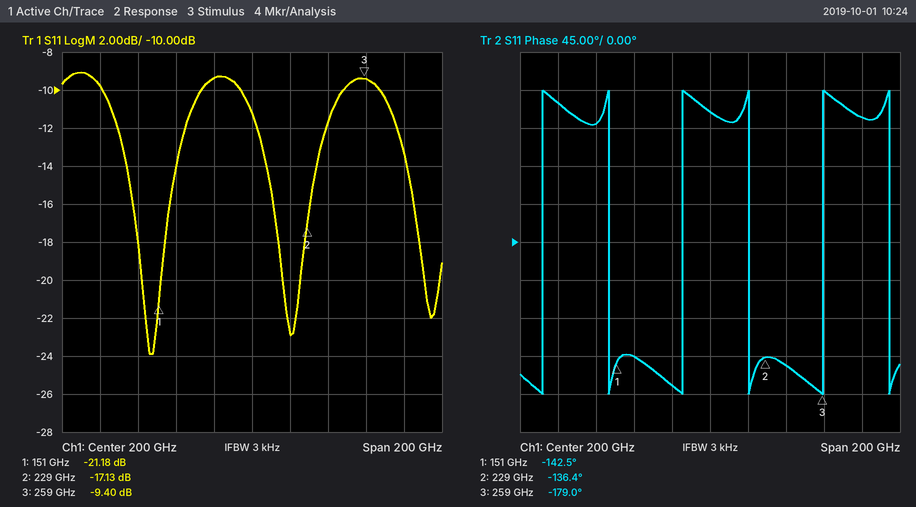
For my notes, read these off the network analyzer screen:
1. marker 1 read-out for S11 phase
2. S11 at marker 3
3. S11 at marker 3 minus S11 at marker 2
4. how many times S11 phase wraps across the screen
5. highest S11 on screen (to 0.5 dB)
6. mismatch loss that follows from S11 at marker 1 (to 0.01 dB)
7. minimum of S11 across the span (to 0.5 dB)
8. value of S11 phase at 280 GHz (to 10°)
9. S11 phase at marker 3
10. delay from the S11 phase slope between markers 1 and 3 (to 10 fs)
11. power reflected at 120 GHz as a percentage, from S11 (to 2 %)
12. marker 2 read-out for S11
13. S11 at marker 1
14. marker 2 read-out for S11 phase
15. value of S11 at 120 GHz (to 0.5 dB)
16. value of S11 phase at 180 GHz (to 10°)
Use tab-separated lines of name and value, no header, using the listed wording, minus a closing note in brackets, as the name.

marker 1 read-out for S11 phase	-142.5°
S11 at marker 3	-9.40 dB
S11 at marker 3 minus S11 at marker 2	7.73 dB
how many times S11 phase wraps across the screen	6
highest S11 on screen	-9.0 dB
mismatch loss that follows from S11 at marker 1	0.03 dB
minimum of S11 across the span	-24.0 dB
value of S11 phase at 280 GHz	150°
S11 phase at marker 3	-179.0°
delay from the S11 phase slope between markers 1 and 3	940 fs
power reflected at 120 GHz as a percentage, from S11	10 %
marker 2 read-out for S11	-17.13 dB
S11 at marker 1	-21.18 dB
marker 2 read-out for S11 phase	-136.4°
value of S11 at 120 GHz	-10.0 dB
value of S11 phase at 180 GHz	-170°
